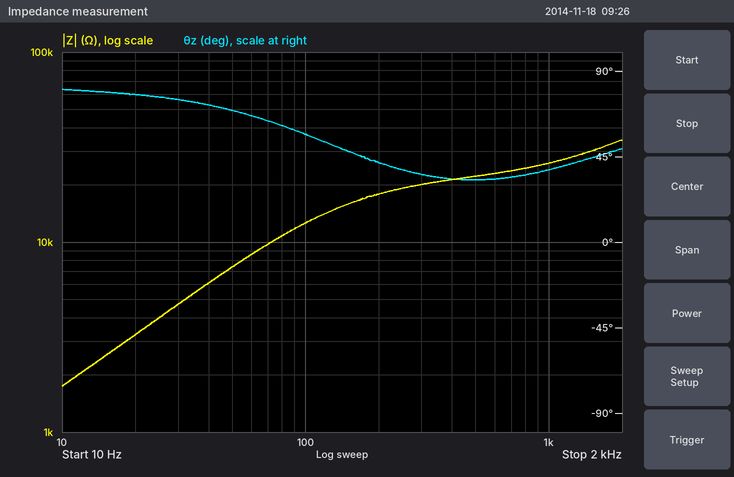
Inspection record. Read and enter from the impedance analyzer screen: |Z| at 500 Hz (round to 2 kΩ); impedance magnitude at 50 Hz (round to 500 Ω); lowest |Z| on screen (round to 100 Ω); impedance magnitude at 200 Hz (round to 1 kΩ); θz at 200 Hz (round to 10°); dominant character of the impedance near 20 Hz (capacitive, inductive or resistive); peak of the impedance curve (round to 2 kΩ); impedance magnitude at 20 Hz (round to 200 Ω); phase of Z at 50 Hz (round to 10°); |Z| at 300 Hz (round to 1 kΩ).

22 kΩ
7.5 kΩ
1.7 kΩ
18 kΩ
40°
inductive
34 kΩ
3.2 kΩ
70°
20 kΩ
